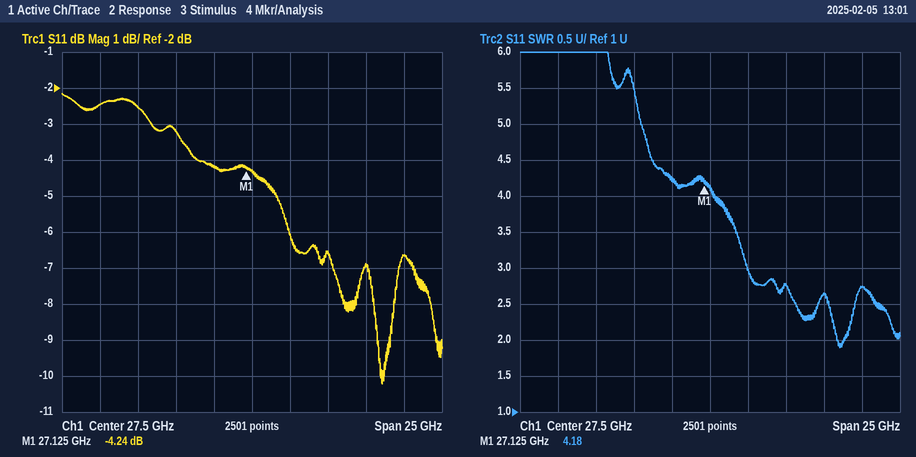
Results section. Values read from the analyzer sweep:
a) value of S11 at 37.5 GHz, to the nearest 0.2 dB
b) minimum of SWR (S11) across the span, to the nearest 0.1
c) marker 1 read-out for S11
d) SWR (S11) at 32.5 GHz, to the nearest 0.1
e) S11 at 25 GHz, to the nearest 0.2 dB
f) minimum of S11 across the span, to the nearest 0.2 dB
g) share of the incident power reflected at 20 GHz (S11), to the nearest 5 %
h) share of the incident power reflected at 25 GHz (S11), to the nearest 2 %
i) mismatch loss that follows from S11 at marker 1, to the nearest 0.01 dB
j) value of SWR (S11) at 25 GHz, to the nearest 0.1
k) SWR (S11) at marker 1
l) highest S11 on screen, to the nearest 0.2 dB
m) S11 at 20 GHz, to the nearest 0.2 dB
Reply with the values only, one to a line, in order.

-6.6 dB
1.9
-4.24 dB
2.8
-4.2 dB
-10.2 dB
55 %
38 %
2.05 dB
4.2
4.18
-2.2 dB
-2.6 dB
